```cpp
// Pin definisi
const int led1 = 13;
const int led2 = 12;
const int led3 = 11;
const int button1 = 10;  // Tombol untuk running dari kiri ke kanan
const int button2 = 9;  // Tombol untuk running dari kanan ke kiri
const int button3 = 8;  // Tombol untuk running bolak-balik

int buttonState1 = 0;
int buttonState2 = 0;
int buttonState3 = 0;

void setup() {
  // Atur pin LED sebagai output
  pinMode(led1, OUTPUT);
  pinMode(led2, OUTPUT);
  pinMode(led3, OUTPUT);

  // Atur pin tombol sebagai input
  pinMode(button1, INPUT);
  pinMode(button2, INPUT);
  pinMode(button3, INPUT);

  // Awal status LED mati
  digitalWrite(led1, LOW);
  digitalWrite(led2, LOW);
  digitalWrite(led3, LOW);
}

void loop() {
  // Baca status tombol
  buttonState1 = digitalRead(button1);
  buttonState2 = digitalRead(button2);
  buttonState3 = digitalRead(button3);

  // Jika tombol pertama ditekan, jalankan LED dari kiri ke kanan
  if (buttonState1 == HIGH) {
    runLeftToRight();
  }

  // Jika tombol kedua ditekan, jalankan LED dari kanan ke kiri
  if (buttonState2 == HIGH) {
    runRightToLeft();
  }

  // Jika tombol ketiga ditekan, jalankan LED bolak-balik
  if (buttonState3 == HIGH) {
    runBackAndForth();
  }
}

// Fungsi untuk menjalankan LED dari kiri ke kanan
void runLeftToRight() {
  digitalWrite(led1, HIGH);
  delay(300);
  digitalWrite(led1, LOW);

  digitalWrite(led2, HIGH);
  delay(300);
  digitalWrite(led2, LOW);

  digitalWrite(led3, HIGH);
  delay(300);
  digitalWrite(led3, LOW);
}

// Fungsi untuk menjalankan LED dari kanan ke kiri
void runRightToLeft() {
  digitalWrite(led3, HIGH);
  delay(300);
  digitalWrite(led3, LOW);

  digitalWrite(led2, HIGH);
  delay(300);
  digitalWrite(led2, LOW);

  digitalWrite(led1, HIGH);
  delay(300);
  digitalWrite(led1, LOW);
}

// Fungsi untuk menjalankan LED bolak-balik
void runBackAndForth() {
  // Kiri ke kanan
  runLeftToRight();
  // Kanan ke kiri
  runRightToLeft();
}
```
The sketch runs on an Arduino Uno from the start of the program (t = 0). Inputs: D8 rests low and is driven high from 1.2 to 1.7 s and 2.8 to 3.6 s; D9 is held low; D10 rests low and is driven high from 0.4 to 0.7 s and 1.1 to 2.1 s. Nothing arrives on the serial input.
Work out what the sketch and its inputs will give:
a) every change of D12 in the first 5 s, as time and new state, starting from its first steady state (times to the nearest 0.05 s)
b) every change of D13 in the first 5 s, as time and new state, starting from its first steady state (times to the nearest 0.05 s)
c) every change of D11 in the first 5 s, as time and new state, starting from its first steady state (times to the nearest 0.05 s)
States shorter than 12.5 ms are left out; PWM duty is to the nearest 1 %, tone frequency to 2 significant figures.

0 s low; 0.7 s high; 1 s low; 1.6 s high; 1.9 s low; 2.5 s high; 2.8 s low; 3.4 s high; 3.7 s low
0 s low; 0.4 s high; 0.7 s low; 1.3 s high; 1.6 s low; 2.2 s high; 2.5 s low; 3.7 s high; 4 s low
0 s low; 1 s high; 1.3 s low; 1.9 s high; 2.2 s low; 2.8 s high; 3.4 s low
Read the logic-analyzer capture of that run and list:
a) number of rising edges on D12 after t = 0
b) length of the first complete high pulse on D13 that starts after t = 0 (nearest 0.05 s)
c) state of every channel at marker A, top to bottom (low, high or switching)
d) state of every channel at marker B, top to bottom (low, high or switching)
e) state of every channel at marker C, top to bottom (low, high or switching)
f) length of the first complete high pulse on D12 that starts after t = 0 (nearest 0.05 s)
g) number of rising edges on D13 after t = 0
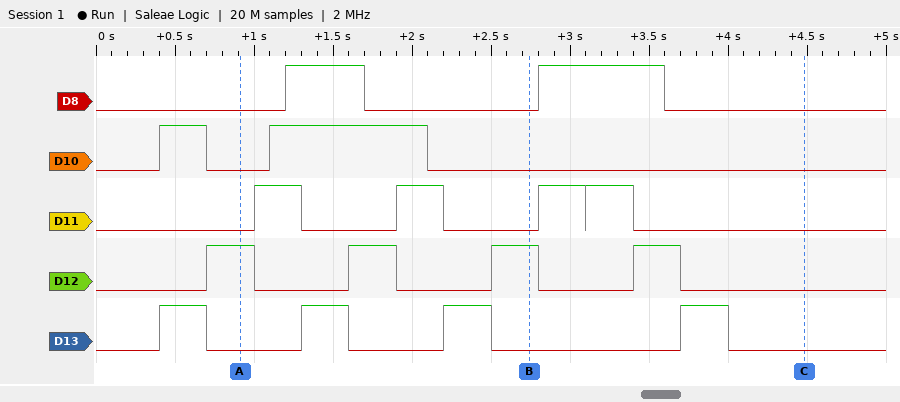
4
0.30 s
D8 low, D10 low, D11 low, D12 high, D13 low
D8 low, D10 low, D11 low, D12 high, D13 low
D8 low, D10 low, D11 low, D12 low, D13 low
0.30 s
4
